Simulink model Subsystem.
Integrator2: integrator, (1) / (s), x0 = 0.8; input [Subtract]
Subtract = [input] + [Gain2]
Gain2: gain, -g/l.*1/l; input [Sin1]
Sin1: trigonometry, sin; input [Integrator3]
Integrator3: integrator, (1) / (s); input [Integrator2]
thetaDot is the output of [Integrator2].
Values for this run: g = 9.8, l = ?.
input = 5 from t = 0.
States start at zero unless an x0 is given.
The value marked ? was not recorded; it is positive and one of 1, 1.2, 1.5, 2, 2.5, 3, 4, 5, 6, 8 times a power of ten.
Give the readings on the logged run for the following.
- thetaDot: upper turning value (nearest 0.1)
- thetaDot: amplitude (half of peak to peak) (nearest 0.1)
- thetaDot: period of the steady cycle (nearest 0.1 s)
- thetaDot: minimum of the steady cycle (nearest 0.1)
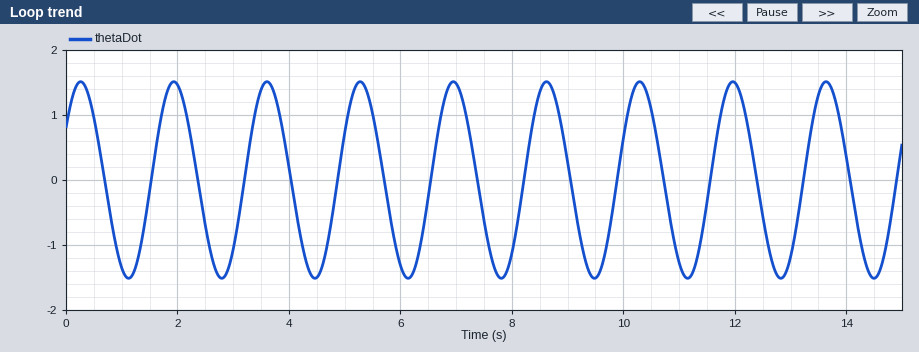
1.5
1.5
1.7 s
-1.5
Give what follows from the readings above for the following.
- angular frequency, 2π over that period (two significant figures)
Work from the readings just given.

3.7 rad/s
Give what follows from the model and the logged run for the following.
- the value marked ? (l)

0.8
